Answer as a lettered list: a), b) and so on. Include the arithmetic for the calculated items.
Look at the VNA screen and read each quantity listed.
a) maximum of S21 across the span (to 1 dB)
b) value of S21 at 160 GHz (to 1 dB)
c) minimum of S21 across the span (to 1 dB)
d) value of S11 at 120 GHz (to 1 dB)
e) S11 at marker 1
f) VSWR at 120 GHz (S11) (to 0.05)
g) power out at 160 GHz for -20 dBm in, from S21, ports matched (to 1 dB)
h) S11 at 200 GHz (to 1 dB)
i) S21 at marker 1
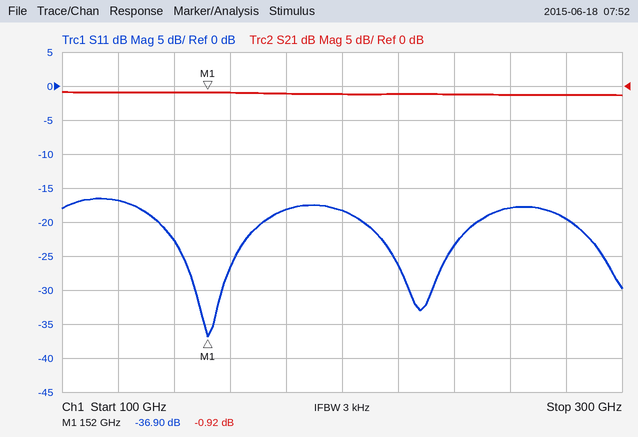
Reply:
a) -1 dB
b) -1 dB
c) -1 dB
d) -17 dB
e) -36.90 dB
f) |Γ| = 10^(-17/20) = 0.1413; VSWR = (1 + 0.1413)/(1 − 0.1413) ≈ 1.33, so 1.35 to the nearest 0.05
g) -20 dBm + (-1 dB) = -21 dBm
h) -18 dB
i) -0.92 dB
